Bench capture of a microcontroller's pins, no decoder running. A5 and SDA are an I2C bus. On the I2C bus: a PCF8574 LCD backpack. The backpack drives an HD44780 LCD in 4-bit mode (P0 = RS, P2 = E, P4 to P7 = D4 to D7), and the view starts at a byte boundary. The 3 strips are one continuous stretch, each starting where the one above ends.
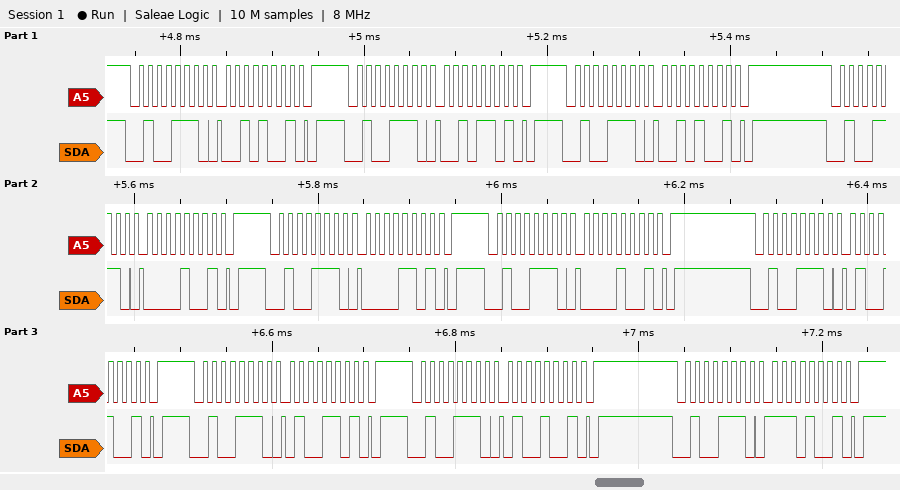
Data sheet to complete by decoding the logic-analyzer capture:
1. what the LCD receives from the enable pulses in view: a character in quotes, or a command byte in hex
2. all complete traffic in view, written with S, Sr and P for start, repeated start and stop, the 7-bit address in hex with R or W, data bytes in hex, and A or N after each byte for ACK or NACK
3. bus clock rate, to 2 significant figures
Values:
' '
S 27W A 29 A P S 27W A 2D A P S 27W A 29 A P S 27W A 09 A P S 27W A 0D A P S 27W A 09 A P S 27W A 49 A P S 27W A 4D A P S 27W A 49 A P S 27W A E9 A P
100 kHz
